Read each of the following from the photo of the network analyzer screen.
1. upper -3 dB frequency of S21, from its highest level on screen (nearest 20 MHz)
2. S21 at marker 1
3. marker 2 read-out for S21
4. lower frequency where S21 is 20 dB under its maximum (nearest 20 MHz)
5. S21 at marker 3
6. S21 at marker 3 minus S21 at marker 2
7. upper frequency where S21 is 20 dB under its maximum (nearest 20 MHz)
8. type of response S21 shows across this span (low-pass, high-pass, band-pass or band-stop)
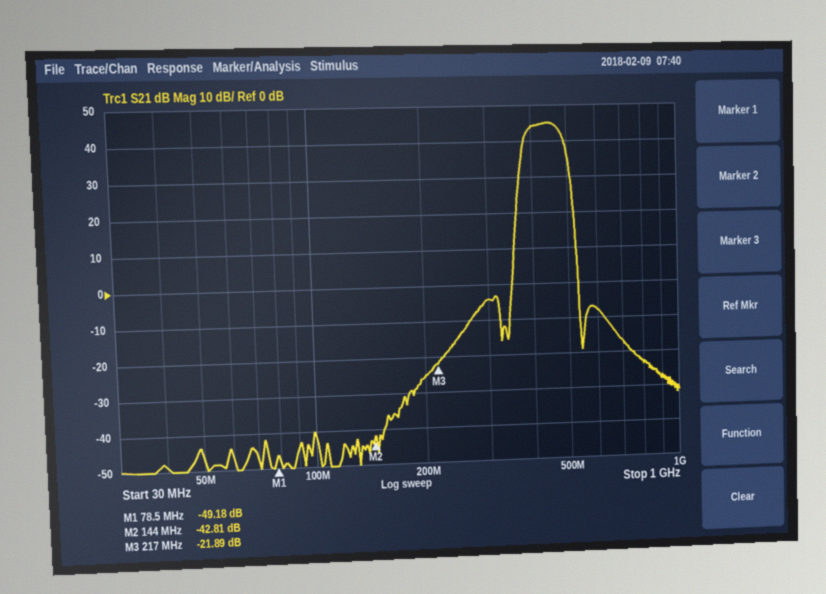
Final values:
480 MHz
-49.18 dB
-42.81 dB
360 MHz
-21.89 dB
20.92 dB
520 MHz
band-pass
